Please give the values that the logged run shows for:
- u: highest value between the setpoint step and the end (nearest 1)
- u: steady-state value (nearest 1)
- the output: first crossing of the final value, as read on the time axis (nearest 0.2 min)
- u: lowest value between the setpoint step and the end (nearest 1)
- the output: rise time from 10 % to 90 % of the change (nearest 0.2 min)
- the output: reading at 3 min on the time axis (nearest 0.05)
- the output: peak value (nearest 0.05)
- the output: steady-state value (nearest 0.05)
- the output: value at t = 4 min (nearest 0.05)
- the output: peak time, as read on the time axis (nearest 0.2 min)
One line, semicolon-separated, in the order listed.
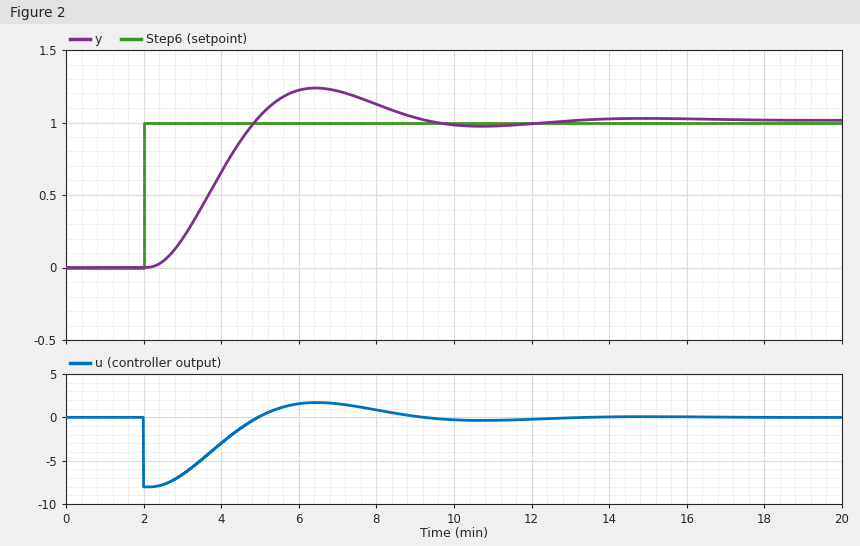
2; 0; 4.8 min; -8; 1.8 min; 0.20; 1.25; 1.00; 0.65; 6.4 min
